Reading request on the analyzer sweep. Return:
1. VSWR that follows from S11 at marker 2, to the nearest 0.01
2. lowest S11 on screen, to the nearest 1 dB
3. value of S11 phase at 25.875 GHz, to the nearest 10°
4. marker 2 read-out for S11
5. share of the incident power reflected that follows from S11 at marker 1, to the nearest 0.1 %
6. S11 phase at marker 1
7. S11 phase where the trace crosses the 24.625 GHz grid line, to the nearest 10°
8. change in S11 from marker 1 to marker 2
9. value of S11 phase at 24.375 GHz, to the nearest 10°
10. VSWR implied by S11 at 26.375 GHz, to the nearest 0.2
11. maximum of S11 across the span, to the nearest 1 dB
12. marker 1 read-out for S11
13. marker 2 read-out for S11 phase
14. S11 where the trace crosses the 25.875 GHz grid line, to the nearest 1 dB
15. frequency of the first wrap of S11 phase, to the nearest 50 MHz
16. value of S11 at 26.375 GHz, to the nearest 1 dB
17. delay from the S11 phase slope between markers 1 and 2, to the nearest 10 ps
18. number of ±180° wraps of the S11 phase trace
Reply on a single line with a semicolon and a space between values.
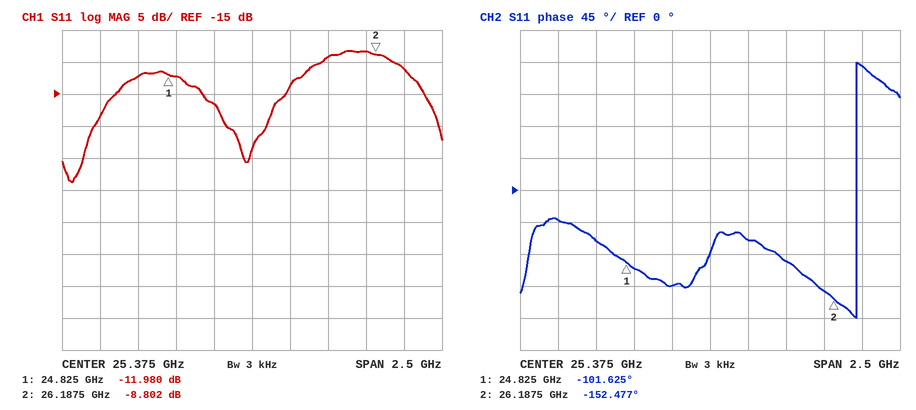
2.14; -29 dB; -100°; -8.802 dB; 6.3 %; -101.625°; -70°; 3.178 dB; -40°; 1.8; -8 dB; -11.980 dB; -152.477°; -9 dB; 26.35 GHz; -11 dB; 100 ps; 1
